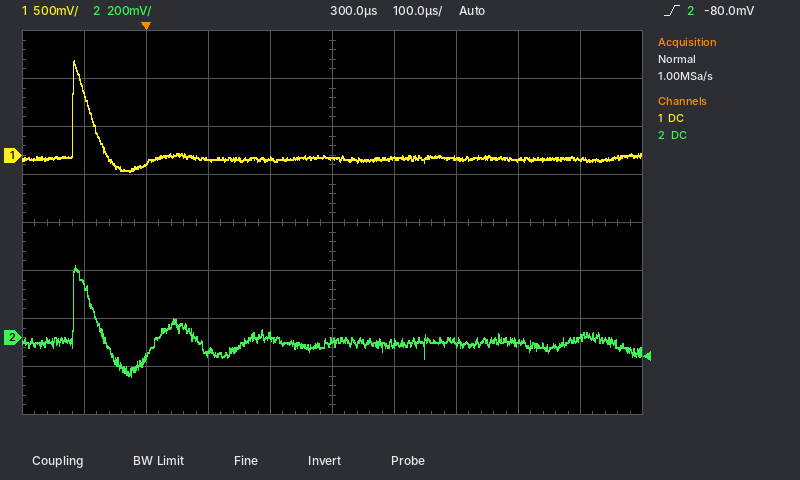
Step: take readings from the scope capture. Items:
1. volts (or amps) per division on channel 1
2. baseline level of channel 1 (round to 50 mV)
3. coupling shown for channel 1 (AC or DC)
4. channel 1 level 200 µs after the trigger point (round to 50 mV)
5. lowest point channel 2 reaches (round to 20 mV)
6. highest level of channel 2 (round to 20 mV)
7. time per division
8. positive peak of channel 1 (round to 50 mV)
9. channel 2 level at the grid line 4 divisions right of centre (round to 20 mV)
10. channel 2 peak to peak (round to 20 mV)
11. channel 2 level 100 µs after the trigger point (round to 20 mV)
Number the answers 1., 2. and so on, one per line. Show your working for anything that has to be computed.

1. 500 mV
2. -50 mV
3. DC
4. -50 mV
5. -160 mV
6. 300 mV
7. 100 µs
8. 1.00 V
9. 0 mV
10. 300 mV − (-160 mV) = 460 mV
11. -60 mV
